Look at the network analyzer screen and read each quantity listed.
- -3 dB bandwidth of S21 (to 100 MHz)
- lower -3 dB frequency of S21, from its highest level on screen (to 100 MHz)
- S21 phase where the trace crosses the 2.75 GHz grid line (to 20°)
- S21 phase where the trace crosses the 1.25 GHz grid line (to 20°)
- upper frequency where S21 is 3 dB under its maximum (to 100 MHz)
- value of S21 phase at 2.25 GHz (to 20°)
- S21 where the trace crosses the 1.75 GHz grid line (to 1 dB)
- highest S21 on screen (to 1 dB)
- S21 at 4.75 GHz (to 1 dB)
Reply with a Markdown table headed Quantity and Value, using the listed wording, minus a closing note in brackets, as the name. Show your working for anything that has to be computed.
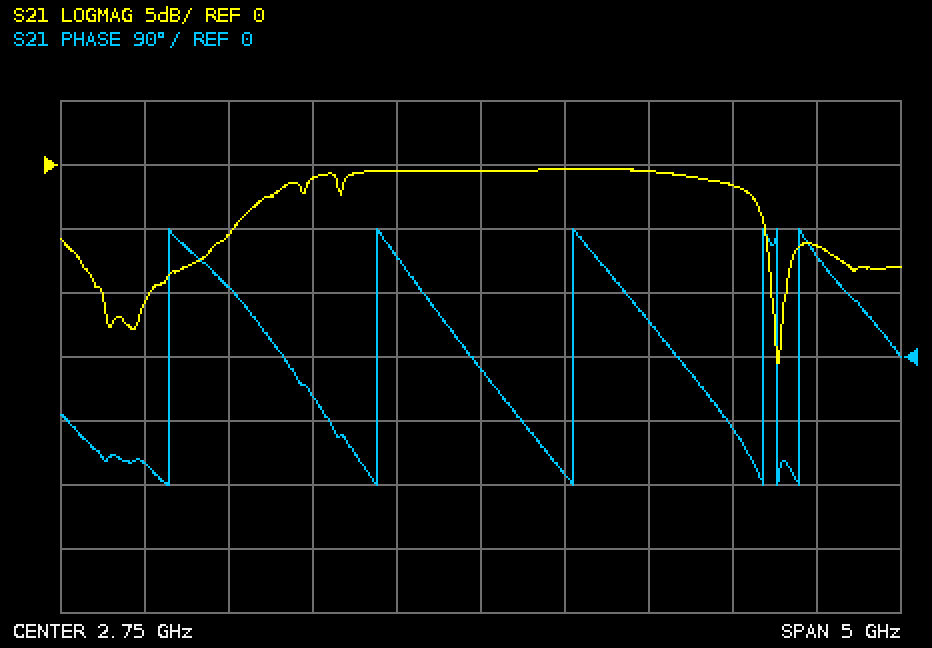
| Quantity | Value |
|---|---|
| -3 dB bandwidth of S21 | 4.4 GHz − 1.4 GHz = 3.0 GHz |
| lower -3 dB frequency of S21, from its highest level on screen | 1.4 GHz |
| S21 phase where the trace crosses the 2.75 GHz grid line | -20° |
| S21 phase where the trace crosses the 1.25 GHz grid line | 100° |
| upper frequency where S21 is 3 dB under its maximum | 4.4 GHz |
| value of S21 phase at 2.25 GHz | 140° |
| S21 where the trace crosses the 1.75 GHz grid line | -1 dB |
| highest S21 on screen | 0 dB |
| S21 at 4.75 GHz | -6 dB |
